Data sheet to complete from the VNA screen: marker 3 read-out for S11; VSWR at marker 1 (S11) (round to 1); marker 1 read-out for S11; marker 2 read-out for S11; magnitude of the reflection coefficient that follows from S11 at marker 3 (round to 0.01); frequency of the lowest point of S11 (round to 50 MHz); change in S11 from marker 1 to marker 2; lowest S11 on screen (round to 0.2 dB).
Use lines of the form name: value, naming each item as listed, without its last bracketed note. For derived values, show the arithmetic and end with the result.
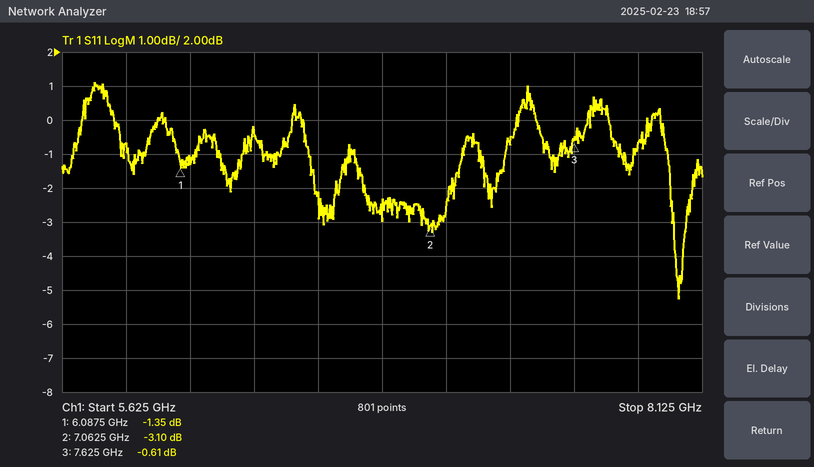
marker 3 read-out for S11: -0.61 dB
VSWR at marker 1 (S11): (1 + 0.8561)/(1 − 0.8561) ≈ 13
marker 1 read-out for S11: -1.35 dB
marker 2 read-out for S11: -3.10 dB
magnitude of the reflection coefficient that follows from S11 at marker 3: 10^(-0.61/20) ≈ 0.93
frequency of the lowest point of S11: 8.05 GHz
change in S11 from marker 1 to marker 2: -3.1 − (-1.35) = -1.75 dB
lowest S11 on screen: -5.2 dB
